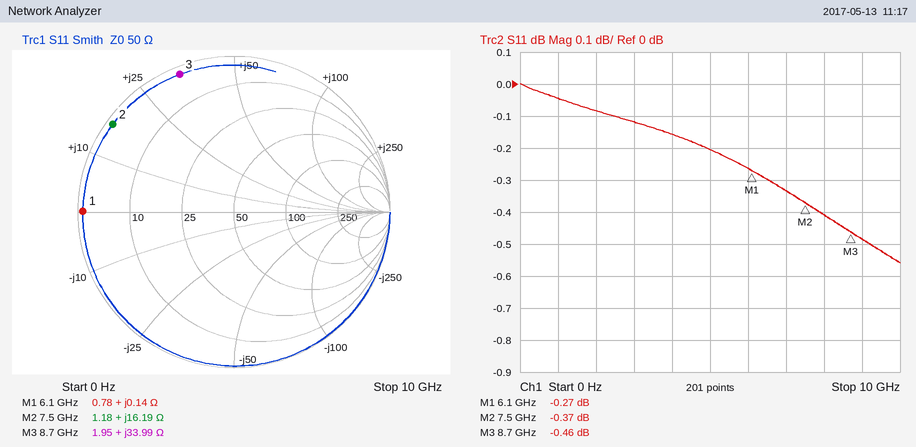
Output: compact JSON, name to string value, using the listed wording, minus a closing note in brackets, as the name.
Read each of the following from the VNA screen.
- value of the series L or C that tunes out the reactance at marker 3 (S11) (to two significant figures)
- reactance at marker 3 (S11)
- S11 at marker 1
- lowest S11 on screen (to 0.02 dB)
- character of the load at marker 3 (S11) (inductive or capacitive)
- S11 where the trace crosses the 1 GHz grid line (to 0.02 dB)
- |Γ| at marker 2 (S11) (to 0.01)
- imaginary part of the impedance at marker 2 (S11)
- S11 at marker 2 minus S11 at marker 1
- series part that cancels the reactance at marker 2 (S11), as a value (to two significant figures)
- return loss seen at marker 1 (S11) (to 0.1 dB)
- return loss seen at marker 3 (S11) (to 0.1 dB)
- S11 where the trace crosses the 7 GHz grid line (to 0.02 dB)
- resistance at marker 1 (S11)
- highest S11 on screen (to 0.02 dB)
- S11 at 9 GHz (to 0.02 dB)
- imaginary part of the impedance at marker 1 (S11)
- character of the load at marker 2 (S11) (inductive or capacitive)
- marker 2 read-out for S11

{"value of the series L or C that tunes out the reactance at marker 3 (S11)": "540 fF", "reactance at marker 3": "+33.99 Ω", "S11 at marker 1": "-0.27 dB", "lowest S11 on screen": "-0.56 dB", "character of the load at marker 3 (S11)": "inductive", "S11 where the trace crosses the 1 GHz grid line": "-0.04 dB", "|Γ| at marker 2 (S11)": "0.96", "imaginary part of the impedance at marker 2": "+16.19 Ω", "S11 at marker 2 minus S11 at marker 1": "-0.10 dB", "series part that cancels the reactance at marker 2 (S11), as a value": "1.3 pF", "return loss seen at marker 1 (S11)": "0.3 dB", "return loss seen at marker 3 (S11)": "0.5 dB", "S11 where the trace crosses the 7 GHz grid line": "-0.34 dB", "resistance at marker 1": "0.78 Ω", "highest S11 on screen": "0.00 dB", "S11 at 9 GHz": "-0.48 dB", "imaginary part of the impedance at marker 1": "+0.14 Ω", "character of the load at marker 2 (S11)": "inductive", "marker 2 read-out for S11": "-0.37 dB"}
